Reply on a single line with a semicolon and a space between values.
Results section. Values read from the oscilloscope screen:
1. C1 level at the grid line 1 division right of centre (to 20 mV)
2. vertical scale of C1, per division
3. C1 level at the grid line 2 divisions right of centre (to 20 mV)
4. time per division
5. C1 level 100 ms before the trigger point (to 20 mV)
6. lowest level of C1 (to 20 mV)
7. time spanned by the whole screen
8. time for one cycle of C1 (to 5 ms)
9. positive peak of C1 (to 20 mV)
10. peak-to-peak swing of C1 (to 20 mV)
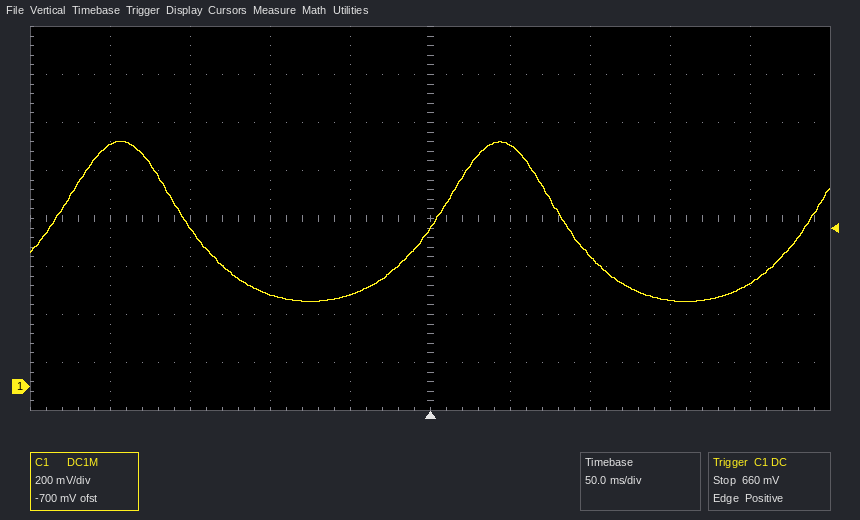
1.00 V; 200 mV; 540 mV; 50 ms; 380 mV; 360 mV; 500 ms; 235 ms; 1.02 V; 660 mV
